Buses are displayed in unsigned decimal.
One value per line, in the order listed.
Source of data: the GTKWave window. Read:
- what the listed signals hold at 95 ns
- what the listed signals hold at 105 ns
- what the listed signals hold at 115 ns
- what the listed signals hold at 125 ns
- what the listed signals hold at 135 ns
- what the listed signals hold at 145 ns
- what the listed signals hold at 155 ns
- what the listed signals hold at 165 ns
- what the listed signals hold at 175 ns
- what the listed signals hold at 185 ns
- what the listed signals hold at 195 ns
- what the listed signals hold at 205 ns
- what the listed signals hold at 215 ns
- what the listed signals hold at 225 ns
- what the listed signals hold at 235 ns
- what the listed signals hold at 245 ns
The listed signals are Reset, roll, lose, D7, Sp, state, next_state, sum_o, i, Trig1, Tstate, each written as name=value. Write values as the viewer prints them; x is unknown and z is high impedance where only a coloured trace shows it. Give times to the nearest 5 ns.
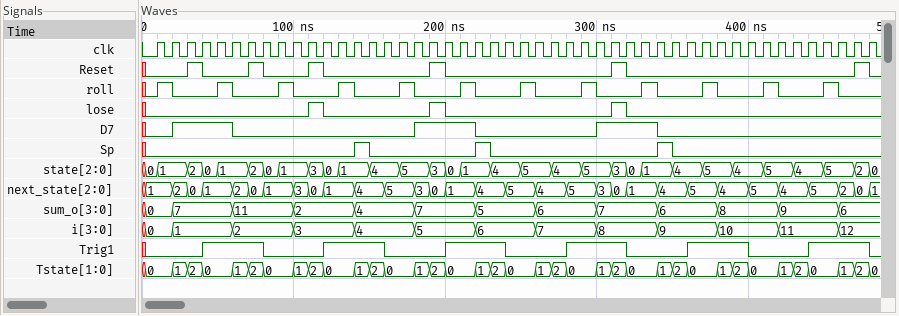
Reset=0, roll=1, lose=0, D7=0, Sp=0, state=1, next_state=1, sum_o=11, i=2, Trig1=0, Tstate=0
Reset=0, roll=0, lose=0, D7=0, Sp=0, state=1, next_state=3, sum_o=2, i=3, Trig1=0, Tstate=1
Reset=1, roll=0, lose=1, D7=0, Sp=0, state=3, next_state=0, sum_o=2, i=3, Trig1=0, Tstate=2
Reset=0, roll=0, lose=0, D7=0, Sp=0, state=0, next_state=1, sum_o=2, i=3, Trig1=1, Tstate=0
Reset=0, roll=1, lose=0, D7=0, Sp=0, state=1, next_state=1, sum_o=2, i=3, Trig1=1, Tstate=0
Reset=0, roll=0, lose=0, D7=0, Sp=1, state=1, next_state=4, sum_o=4, i=4, Trig1=1, Tstate=1
Reset=0, roll=0, lose=0, D7=0, Sp=0, state=4, next_state=4, sum_o=4, i=4, Trig1=1, Tstate=2
Reset=0, roll=0, lose=0, D7=0, Sp=0, state=4, next_state=5, sum_o=4, i=4, Trig1=0, Tstate=0
Reset=0, roll=1, lose=0, D7=0, Sp=0, state=5, next_state=5, sum_o=4, i=4, Trig1=0, Tstate=0
Reset=0, roll=0, lose=0, D7=1, Sp=0, state=5, next_state=3, sum_o=7, i=5, Trig1=0, Tstate=1
Reset=1, roll=0, lose=1, D7=1, Sp=0, state=3, next_state=0, sum_o=7, i=5, Trig1=0, Tstate=2
Reset=0, roll=0, lose=0, D7=1, Sp=0, state=0, next_state=1, sum_o=7, i=5, Trig1=1, Tstate=0
Reset=0, roll=1, lose=0, D7=1, Sp=0, state=1, next_state=1, sum_o=7, i=5, Trig1=1, Tstate=0
Reset=0, roll=0, lose=0, D7=0, Sp=1, state=1, next_state=4, sum_o=5, i=6, Trig1=1, Tstate=1
Reset=0, roll=0, lose=0, D7=0, Sp=0, state=4, next_state=4, sum_o=5, i=6, Trig1=1, Tstate=2
Reset=0, roll=0, lose=0, D7=0, Sp=0, state=4, next_state=5, sum_o=5, i=6, Trig1=0, Tstate=0
